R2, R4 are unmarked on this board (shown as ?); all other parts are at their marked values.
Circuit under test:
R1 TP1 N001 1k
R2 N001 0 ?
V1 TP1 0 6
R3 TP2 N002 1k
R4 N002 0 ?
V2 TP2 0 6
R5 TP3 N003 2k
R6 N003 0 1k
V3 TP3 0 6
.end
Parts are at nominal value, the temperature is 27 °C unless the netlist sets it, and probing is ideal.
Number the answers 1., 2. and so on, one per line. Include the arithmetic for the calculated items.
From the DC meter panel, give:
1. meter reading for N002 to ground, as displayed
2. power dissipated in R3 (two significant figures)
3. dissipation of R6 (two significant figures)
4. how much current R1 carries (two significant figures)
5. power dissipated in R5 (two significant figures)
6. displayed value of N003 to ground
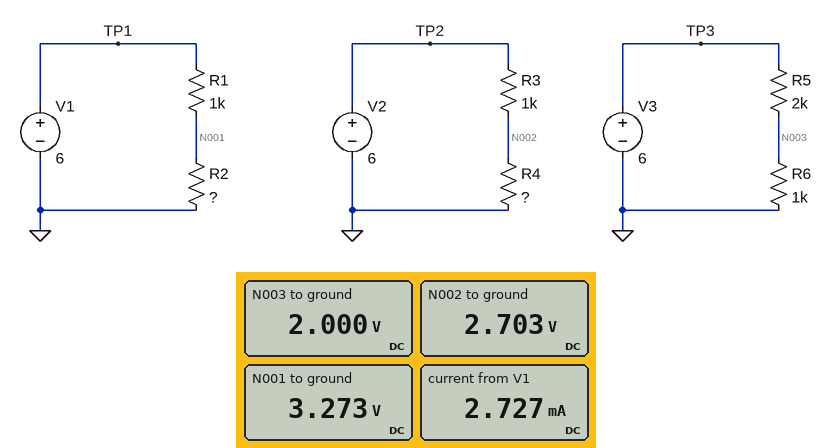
1. 2.703 V
2. (6 V - 2.703 V)^2 / 1 kΩ = 11 mW
3. (2 V)^2 / 1 kΩ = 4.0 mW
4. (6 V - 3.273 V) / 1 kΩ = 2.7 mA
5. (6 V - 2 V)^2 / 2 kΩ = 8.0 mW
6. 2.000 V
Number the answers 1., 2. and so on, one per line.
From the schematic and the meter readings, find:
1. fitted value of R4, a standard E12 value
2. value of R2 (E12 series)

1. 820 Ω
2. 1.2 kΩ
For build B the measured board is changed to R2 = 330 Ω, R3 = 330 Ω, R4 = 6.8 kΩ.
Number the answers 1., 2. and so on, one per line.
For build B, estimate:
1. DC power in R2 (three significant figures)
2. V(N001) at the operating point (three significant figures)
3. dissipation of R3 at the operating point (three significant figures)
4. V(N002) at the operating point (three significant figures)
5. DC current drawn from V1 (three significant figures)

1. 6.72 mW
2. 1.49 V
3. 234 µW
4. 5.72 V
5. 4.51 mA
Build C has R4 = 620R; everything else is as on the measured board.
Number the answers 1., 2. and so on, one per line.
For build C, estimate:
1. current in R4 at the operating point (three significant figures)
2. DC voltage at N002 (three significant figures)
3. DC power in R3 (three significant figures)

1. 3.70 mA
2. 2.30 V
3. 13.7 mW
